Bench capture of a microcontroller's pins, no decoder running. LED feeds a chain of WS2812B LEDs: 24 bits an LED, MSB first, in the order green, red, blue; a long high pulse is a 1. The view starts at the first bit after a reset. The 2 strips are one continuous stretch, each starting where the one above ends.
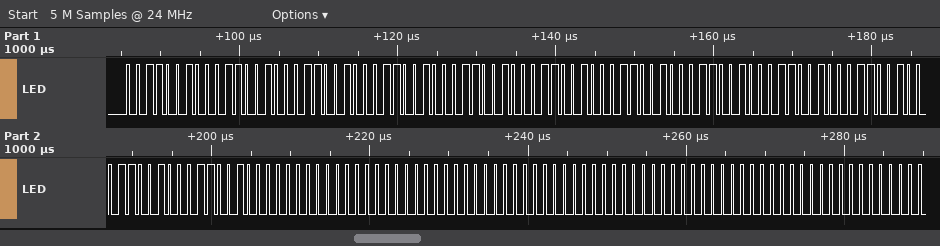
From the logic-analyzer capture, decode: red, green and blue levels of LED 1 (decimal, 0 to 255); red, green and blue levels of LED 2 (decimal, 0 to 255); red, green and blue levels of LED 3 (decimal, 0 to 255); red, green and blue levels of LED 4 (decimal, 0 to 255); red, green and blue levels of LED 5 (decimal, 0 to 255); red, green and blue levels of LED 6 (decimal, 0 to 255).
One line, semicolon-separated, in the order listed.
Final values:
50, 50, 50; 50, 50, 50; 50, 50, 50; 50, 50, 50; 0, 0, 0; 0, 0, 0
